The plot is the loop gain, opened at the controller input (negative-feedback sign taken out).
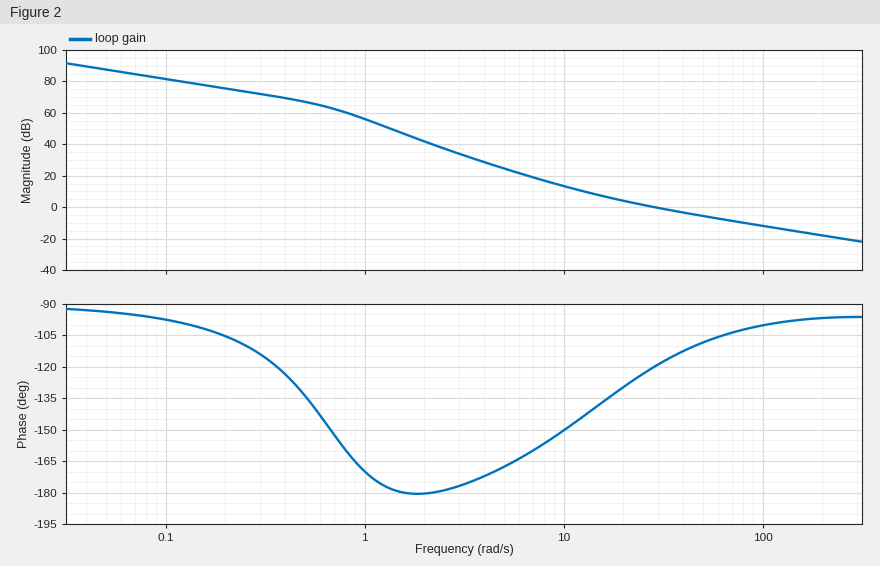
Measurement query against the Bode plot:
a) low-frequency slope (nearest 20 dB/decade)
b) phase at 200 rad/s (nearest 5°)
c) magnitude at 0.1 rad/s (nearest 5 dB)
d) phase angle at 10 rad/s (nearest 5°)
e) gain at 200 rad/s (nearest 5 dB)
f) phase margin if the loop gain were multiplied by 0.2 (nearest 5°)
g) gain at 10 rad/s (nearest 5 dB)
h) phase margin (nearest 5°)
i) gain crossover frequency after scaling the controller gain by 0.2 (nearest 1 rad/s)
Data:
-20 dB/decade
-95°
80 dB
-150°
-20 dB
30°
15 dB
60°
10 rad/s
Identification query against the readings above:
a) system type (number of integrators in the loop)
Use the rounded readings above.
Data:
1
